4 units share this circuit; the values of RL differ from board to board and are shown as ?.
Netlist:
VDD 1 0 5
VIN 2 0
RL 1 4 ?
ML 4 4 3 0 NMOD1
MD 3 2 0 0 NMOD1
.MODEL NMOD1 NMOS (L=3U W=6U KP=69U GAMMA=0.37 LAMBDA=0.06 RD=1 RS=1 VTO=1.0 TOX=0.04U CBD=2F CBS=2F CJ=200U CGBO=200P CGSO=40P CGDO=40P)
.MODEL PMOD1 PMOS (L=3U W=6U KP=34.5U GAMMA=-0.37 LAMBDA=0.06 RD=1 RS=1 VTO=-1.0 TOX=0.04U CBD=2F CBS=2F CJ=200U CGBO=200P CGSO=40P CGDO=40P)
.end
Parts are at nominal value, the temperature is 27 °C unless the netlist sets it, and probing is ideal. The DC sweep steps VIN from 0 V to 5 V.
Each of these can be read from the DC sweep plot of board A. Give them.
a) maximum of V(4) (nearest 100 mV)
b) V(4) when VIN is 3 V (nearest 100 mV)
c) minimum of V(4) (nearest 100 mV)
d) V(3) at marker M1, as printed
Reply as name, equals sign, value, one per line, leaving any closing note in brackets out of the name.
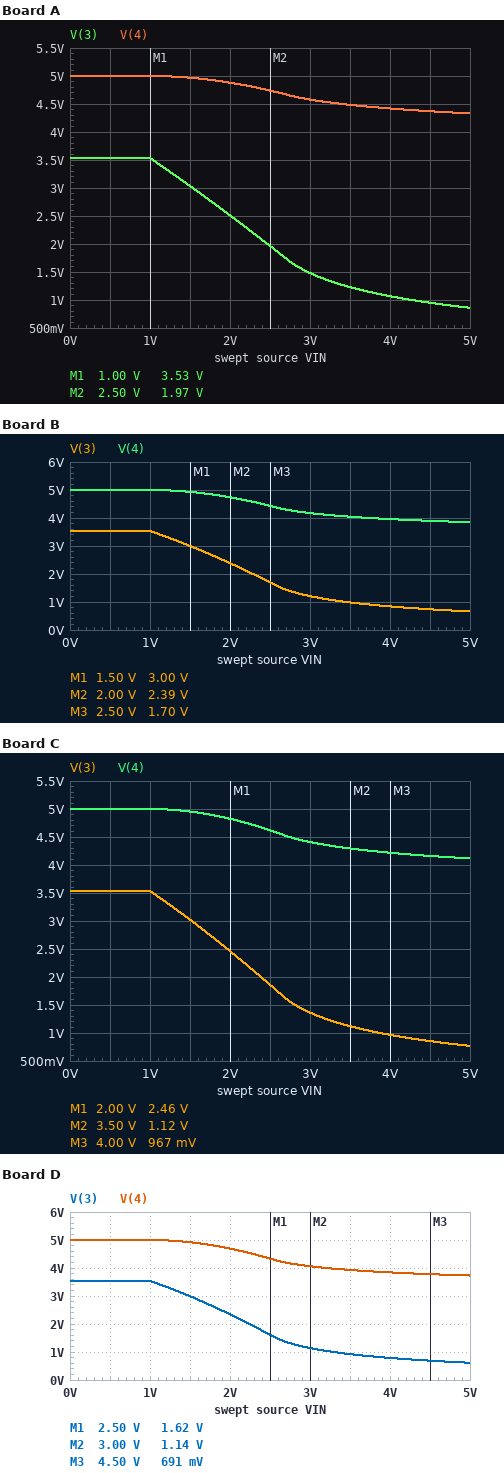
maximum of V(4) = 5.0 V
V(4) when VIN is 3 V = 4.6 V
minimum of V(4) = 4.3 V
V(3) at marker M1, as printed = 3.53 V
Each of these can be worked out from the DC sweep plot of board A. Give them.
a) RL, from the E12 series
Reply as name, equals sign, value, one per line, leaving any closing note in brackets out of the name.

RL, from the E12 series = 1.5 kΩ
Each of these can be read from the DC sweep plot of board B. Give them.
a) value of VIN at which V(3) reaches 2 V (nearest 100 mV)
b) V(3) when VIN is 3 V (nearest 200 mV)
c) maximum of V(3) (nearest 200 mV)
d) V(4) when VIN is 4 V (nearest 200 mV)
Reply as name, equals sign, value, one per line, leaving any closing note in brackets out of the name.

value of VIN at which V(3) reaches 2 V = 2.3 V
V(3) when VIN is 3 V = 1.2 V
maximum of V(3) = 3.6 V
V(4) when VIN is 4 V = 4.0 V
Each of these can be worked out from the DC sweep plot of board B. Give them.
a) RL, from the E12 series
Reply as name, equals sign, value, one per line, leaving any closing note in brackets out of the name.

RL, from the E12 series = 3.3 kΩ
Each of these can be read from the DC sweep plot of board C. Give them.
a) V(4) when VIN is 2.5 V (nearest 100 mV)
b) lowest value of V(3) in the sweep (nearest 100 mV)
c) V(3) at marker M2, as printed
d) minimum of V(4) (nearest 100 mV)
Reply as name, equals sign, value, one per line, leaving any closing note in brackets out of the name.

V(4) when VIN is 2.5 V = 4.6 V
lowest value of V(3) in the sweep = 800 mV
V(3) at marker M2, as printed = 1.12 V
minimum of V(4) = 4.1 V
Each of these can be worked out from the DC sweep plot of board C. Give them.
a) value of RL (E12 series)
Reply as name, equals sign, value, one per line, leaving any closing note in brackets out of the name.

value of RL = 2.2 kΩ
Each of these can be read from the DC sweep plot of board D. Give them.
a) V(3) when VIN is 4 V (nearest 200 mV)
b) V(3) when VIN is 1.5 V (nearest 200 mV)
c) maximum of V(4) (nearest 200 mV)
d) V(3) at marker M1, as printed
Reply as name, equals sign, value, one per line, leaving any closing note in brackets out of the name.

V(3) when VIN is 4 V = 800 mV
V(3) when VIN is 1.5 V = 3.0 V
maximum of V(4) = 5.0 V
V(3) at marker M1, as printed = 1.62 V
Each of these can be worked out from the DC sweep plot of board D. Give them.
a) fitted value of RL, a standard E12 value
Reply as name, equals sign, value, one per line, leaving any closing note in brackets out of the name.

fitted value of RL, a standard E12 value = 3.9 kΩ
